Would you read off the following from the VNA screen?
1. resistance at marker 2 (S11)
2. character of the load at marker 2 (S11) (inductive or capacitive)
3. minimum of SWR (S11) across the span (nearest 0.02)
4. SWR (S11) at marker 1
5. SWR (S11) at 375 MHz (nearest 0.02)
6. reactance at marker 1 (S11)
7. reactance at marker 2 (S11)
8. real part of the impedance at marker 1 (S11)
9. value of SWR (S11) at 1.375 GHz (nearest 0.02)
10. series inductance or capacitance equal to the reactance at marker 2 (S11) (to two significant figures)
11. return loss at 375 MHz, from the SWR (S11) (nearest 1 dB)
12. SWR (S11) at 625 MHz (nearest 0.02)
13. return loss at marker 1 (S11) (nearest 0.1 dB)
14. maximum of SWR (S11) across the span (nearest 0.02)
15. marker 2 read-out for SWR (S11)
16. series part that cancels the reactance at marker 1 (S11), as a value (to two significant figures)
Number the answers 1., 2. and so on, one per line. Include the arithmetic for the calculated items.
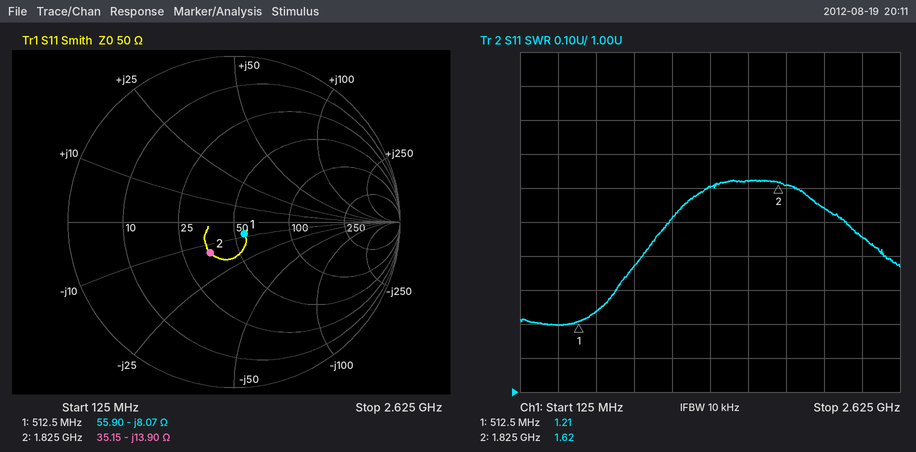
1. 35.15 Ω
2. capacitive
3. 1.20
4. 1.21
5. 1.20
6. -8.07 Ω
7. -13.90 Ω
8. 55.90 Ω
9. 1.60
10. C = 1/(2π × 1.825 GHz × 13.9 Ω) ≈ 6.3 pF
11. −20 log10((1.2 − 1)/(1.2 + 1)) ≈ 21 dB
12. 1.24
13. 20.5 dB
14. 1.62
15. 1.62
16. L = 8.07 Ω/(2π × 512.5 MHz) ≈ 2.5 nH
